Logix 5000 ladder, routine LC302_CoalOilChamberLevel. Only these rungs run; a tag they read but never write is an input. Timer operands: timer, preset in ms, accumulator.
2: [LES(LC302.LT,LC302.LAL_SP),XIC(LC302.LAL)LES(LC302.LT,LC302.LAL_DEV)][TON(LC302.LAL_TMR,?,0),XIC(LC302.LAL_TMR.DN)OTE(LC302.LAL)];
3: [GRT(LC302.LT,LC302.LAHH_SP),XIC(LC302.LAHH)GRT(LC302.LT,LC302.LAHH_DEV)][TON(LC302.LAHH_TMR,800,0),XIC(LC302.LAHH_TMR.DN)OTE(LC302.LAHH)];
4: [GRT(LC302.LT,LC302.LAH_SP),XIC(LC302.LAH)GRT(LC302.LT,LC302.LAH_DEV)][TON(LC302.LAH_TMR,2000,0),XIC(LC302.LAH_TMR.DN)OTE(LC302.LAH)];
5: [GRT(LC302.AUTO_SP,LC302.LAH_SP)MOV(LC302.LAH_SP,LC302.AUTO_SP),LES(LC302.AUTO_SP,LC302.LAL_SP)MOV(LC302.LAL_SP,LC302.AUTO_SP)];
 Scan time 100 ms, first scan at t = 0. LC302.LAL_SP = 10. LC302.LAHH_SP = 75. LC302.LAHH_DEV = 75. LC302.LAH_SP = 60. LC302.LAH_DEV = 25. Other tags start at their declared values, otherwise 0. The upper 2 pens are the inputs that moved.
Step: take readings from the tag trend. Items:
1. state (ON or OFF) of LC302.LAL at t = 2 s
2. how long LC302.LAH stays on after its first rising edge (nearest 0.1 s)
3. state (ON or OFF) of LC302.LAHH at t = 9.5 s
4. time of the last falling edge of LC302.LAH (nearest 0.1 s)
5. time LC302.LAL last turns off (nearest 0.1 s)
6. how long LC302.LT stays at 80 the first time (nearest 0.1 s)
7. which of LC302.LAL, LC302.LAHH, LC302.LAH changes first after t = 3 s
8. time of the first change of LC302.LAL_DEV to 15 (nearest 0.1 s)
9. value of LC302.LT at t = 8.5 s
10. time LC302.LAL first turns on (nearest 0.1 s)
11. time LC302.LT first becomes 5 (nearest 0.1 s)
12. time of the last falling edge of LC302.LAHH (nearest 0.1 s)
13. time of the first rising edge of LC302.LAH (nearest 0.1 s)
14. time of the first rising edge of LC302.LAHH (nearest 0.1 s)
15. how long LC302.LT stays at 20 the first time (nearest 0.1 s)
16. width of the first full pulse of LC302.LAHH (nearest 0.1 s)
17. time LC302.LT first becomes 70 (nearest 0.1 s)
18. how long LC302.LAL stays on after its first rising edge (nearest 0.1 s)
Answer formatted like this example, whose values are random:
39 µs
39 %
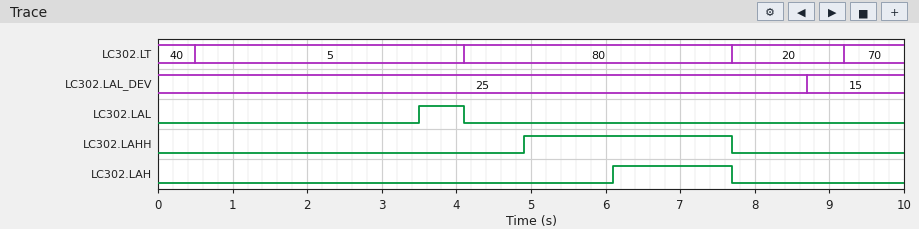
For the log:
OFF
1.6 s
OFF
7.7 s
4.1 s
3.6 s
LC302.LAL
8.7 s
20
3.5 s
0.5 s
7.7 s
6.1 s
4.9 s
1.5 s
2.8 s
9.2 s
0.6 s
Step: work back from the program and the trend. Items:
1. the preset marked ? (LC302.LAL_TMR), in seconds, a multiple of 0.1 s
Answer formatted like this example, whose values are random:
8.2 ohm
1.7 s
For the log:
3.0 s
